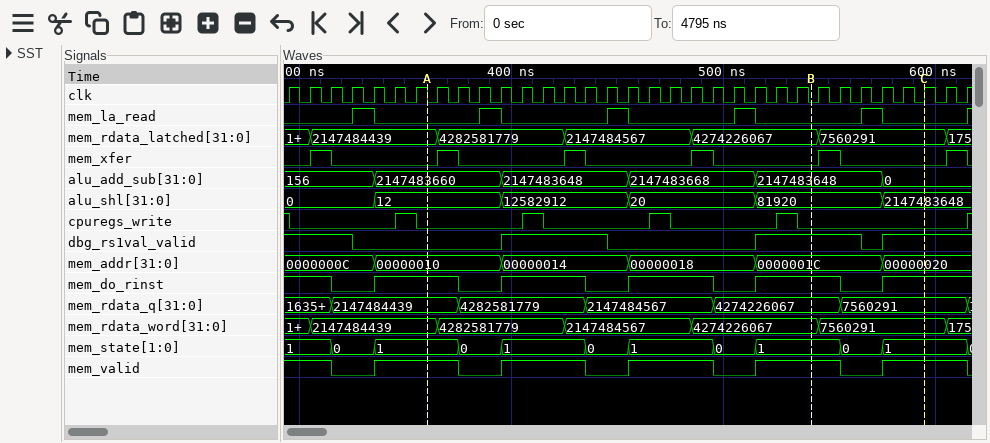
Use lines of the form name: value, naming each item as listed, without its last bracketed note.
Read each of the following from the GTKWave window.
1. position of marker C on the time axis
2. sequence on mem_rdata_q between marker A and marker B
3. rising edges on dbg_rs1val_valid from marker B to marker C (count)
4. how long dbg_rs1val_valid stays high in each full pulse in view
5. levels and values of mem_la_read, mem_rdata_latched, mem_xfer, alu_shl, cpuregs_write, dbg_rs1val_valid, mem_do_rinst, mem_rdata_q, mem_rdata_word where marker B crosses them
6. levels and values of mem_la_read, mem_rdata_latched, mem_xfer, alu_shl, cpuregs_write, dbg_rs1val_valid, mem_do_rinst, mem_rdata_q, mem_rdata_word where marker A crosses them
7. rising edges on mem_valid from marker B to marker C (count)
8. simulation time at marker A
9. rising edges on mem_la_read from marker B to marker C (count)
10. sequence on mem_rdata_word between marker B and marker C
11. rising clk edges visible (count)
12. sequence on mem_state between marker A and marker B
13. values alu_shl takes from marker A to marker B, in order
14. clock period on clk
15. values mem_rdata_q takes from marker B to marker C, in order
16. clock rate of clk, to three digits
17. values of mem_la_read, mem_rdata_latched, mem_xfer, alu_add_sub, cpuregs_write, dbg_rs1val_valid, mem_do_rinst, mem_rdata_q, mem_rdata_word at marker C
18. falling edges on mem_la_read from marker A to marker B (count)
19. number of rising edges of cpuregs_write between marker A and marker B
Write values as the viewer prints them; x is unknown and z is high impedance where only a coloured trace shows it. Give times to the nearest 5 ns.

position of marker C on the time axis: 595 ns
sequence on mem_rdata_q between marker A and marker B: 2147484439, 4282581779, 2147484567, 4274226067
rising edges on dbg_rs1val_valid from marker B to marker C: 1
how long dbg_rs1val_valid stays high in each full pulse in view: 50 ns, 50 ns
levels and values of mem_la_read, mem_rdata_latched, mem_xfer, alu_shl, cpuregs_write, dbg_rs1val_valid, mem_do_rinst, mem_rdata_q, mem_rdata_word where marker B crosses them: mem_la_read=0, mem_rdata_latched=4274226067, mem_xfer=0, alu_shl=81920, cpuregs_write=0, dbg_rs1val_valid=1, mem_do_rinst=1, mem_rdata_q=4274226067, mem_rdata_word=4274226067
levels and values of mem_la_read, mem_rdata_latched, mem_xfer, alu_shl, cpuregs_write, dbg_rs1val_valid, mem_do_rinst, mem_rdata_q, mem_rdata_word where marker A crosses them: mem_la_read=0, mem_rdata_latched=2147484439, mem_xfer=0, alu_shl=12, cpuregs_write=0, dbg_rs1val_valid=0, mem_do_rinst=1, mem_rdata_q=2147484439, mem_rdata_word=2147484439
rising edges on mem_valid from marker B to marker C: 1
simulation time at marker A: 360 ns
rising edges on mem_la_read from marker B to marker C: 1
sequence on mem_rdata_word between marker B and marker C: 4274226067, 7560291
rising clk edges visible: 33
sequence on mem_state between marker A and marker B: 1, 0, 1, 0, 1, 0, 1
values alu_shl takes from marker A to marker B, in order: 12, 12582912, 20, 81920
clock period on clk: 10 ns
values mem_rdata_q takes from marker B to marker C, in order: 4274226067, 7560291
clock rate of clk, to three digits: 100 MHz
values of mem_la_read, mem_rdata_latched, mem_xfer, alu_add_sub, cpuregs_write, dbg_rs1val_valid, mem_do_rinst, mem_rdata_q, mem_rdata_word at marker C: mem_la_read=0, mem_rdata_latched=7560291, mem_xfer=0, alu_add_sub=0, cpuregs_write=0, dbg_rs1val_valid=1, mem_do_rinst=1, mem_rdata_q=7560291, mem_rdata_word=7560291
falling edges on mem_la_read from marker A to marker B: 3
number of rising edges of cpuregs_write between marker A and marker B: 3
